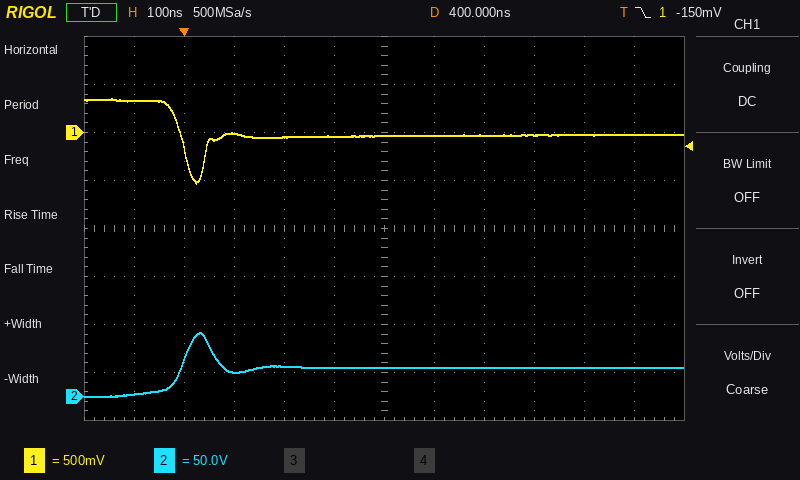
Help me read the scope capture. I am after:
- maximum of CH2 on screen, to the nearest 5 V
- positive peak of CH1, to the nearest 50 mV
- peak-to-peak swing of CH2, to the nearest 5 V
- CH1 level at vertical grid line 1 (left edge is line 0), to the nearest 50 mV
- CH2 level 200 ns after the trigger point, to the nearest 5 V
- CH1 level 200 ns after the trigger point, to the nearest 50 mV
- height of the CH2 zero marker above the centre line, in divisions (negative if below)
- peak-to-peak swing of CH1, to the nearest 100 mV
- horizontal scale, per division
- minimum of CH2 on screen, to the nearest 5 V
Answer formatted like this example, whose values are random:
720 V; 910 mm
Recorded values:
65 V; 350 mV; 65 V; 350 mV; 30 V; -50 mV; -3.5 div; 900 mV; 100 ns; 0 V
